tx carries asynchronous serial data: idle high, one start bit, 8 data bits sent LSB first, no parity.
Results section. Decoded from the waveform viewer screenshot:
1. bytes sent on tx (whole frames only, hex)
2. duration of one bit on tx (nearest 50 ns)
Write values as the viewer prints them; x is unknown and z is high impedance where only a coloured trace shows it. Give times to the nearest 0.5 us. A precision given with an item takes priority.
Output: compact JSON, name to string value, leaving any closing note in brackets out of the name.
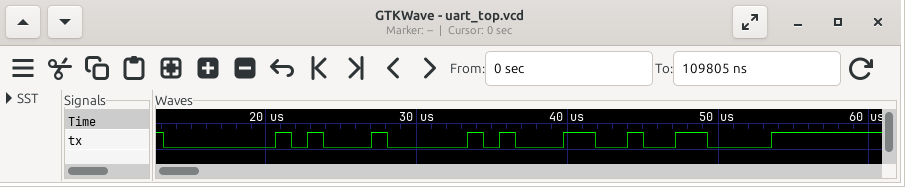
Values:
{"bytes sent on tx": "40, 04, 31, 86", "duration of one bit on tx": "1050 ns"}
